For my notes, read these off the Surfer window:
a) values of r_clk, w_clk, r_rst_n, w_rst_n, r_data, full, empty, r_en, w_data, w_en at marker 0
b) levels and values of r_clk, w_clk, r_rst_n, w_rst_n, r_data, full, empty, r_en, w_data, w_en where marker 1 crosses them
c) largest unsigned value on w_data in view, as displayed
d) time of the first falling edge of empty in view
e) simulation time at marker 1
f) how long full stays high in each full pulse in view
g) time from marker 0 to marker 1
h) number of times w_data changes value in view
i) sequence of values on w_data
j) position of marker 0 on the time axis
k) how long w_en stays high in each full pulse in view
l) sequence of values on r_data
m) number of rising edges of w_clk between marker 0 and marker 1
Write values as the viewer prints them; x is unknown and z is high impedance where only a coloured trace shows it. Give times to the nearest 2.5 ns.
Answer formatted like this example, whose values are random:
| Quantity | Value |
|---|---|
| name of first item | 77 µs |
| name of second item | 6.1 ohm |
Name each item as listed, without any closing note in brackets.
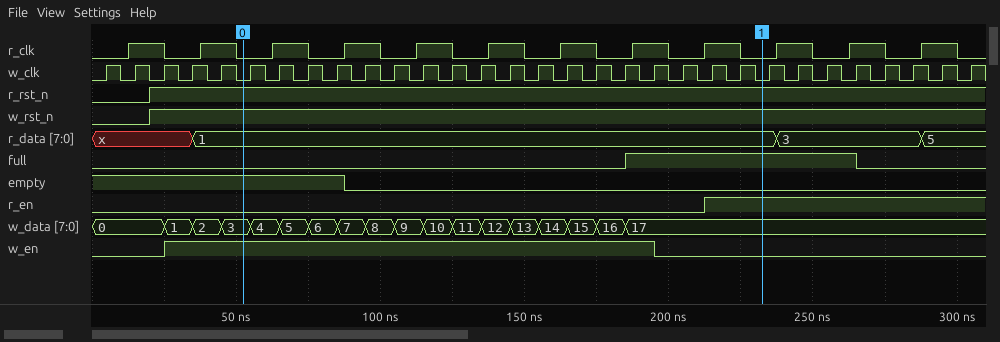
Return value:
| Quantity | Value |
|---|---|
| values of r_clk, w_clk, r_rst_n, w_rst_n, r_data, full, empty, r_en, w_data, w_en at marker 0 | r_clk=0, w_clk=0, r_rst_n=1, w_rst_n=1, r_data=1, full=0, empty=1, r_en=0, w_data=3, w_en=1 |
| levels and values of r_clk, w_clk, r_rst_n, w_rst_n, r_data, full, empty, r_en, w_data, w_en where marker 1 crosses them | r_clk=0, w_clk=0, r_rst_n=1, w_rst_n=1, r_data=1, full=1, empty=0, r_en=1, w_data=17, w_en=0 |
| largest unsigned value on w_data in view, as displayed | 17 |
| time of the first falling edge of empty in view | 87.5 ns |
| simulation time at marker 1 | 232.5 ns |
| how long full stays high in each full pulse in view | 80 ns |
| time from marker 0 to marker 1 | 180 ns |
| number of times w_data changes value in view | 17 |
| sequence of values on w_data | 0, 1, 2, 3, 4, 5, 6, 7, 8, 9, 10, 11, 12, 13, 14, 15, 16, 17 |
| position of marker 0 on the time axis | 52.5 ns |
| how long w_en stays high in each full pulse in view | 170 ns |
| sequence of values on r_data | x, 1, 3, 5 |
| number of rising edges of w_clk between marker 0 and marker 1 | 18 |
